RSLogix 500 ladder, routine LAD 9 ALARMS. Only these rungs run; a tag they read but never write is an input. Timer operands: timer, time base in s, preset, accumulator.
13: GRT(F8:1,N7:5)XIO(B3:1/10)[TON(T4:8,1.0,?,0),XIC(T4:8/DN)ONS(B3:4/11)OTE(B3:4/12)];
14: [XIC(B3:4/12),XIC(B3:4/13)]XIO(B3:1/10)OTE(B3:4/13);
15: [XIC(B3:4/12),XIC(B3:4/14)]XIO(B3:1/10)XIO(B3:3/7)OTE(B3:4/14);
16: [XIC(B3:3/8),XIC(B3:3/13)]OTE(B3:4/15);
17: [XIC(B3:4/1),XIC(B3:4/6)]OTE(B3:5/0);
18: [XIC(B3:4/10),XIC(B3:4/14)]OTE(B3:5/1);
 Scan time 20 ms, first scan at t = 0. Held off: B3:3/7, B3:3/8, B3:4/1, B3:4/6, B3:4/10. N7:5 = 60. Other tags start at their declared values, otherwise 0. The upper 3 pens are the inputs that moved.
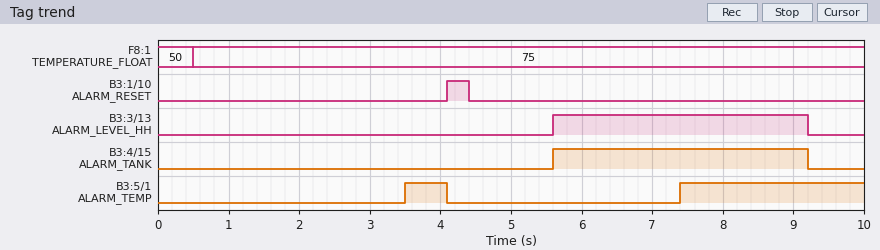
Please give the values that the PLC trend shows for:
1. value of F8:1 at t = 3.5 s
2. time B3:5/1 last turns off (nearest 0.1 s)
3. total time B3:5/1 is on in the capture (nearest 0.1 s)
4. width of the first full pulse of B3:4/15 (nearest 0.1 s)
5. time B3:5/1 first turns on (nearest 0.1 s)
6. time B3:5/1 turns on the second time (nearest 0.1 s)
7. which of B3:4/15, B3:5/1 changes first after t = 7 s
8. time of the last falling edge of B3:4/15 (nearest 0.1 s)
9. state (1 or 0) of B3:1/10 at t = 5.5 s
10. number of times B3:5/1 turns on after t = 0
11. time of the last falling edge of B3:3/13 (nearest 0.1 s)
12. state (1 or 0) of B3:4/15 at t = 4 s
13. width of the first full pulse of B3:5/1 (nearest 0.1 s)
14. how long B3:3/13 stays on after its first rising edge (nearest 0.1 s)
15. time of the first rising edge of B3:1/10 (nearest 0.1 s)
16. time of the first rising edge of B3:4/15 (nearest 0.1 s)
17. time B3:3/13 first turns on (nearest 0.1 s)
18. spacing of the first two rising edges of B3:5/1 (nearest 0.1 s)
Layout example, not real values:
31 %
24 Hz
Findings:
75
4.1 s
3.2 s
3.6 s
3.5 s
7.4 s
B3:5/1
9.2 s
0
2
9.2 s
0
0.6 s
3.6 s
4.1 s
5.6 s
5.6 s
3.9 s
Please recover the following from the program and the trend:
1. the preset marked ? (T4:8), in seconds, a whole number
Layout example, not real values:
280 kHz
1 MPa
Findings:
3 s
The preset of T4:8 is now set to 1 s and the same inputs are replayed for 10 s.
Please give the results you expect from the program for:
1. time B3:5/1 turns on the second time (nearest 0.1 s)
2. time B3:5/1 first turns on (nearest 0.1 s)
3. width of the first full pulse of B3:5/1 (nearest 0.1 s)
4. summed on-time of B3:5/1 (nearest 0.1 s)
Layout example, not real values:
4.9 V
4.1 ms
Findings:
5.4 s
1.5 s
2.6 s
7.2 s
